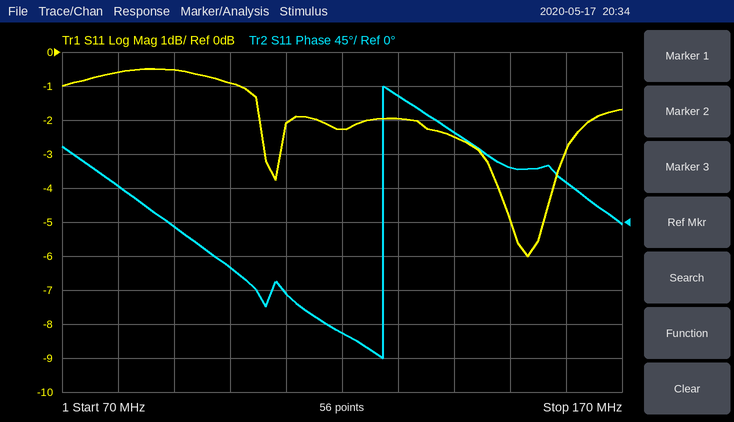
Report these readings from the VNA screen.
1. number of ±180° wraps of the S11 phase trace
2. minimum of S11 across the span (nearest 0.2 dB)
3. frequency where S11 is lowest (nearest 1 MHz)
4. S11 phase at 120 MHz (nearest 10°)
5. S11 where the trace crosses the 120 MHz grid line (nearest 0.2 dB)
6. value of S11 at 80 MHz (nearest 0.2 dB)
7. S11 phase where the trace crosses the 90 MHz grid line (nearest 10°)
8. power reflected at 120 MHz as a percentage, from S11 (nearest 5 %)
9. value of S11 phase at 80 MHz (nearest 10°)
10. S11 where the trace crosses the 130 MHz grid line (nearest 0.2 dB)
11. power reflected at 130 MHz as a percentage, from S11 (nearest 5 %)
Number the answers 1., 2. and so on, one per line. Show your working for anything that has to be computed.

1. 1
2. -6.0 dB
3. 153 MHz
4. -150°
5. -2.2 dB
6. -0.6 dB
7. -10°
8. 10^(-2.2/10) ≈ 60 %
9. 50°
10. -2.0 dB
11. 10^(-2/10) ≈ 63.1 %, so 65 % to the nearest 5 %
